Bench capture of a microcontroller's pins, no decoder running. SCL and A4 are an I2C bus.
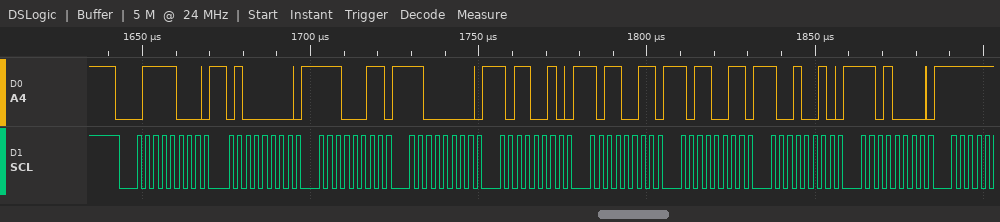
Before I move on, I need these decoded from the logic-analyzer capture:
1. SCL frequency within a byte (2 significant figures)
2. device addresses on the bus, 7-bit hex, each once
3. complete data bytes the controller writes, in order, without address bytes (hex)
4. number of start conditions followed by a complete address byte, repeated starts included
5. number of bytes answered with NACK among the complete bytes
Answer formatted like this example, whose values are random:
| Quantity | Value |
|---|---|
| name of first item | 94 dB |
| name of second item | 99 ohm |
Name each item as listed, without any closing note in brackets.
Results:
| Quantity | Value |
|---|---|
| SCL frequency within a byte | 400 kHz |
| device addresses on the bus, 7-bit hex, each once | 0x3C |
| complete data bytes the controller writes, in order, without address bytes | 40 E3 C0 B2 B3 B3 92 D0 |
| number of start conditions followed by a complete address byte, repeated starts included | 1 |
| number of bytes answered with NACK among the complete bytes | 0 |
